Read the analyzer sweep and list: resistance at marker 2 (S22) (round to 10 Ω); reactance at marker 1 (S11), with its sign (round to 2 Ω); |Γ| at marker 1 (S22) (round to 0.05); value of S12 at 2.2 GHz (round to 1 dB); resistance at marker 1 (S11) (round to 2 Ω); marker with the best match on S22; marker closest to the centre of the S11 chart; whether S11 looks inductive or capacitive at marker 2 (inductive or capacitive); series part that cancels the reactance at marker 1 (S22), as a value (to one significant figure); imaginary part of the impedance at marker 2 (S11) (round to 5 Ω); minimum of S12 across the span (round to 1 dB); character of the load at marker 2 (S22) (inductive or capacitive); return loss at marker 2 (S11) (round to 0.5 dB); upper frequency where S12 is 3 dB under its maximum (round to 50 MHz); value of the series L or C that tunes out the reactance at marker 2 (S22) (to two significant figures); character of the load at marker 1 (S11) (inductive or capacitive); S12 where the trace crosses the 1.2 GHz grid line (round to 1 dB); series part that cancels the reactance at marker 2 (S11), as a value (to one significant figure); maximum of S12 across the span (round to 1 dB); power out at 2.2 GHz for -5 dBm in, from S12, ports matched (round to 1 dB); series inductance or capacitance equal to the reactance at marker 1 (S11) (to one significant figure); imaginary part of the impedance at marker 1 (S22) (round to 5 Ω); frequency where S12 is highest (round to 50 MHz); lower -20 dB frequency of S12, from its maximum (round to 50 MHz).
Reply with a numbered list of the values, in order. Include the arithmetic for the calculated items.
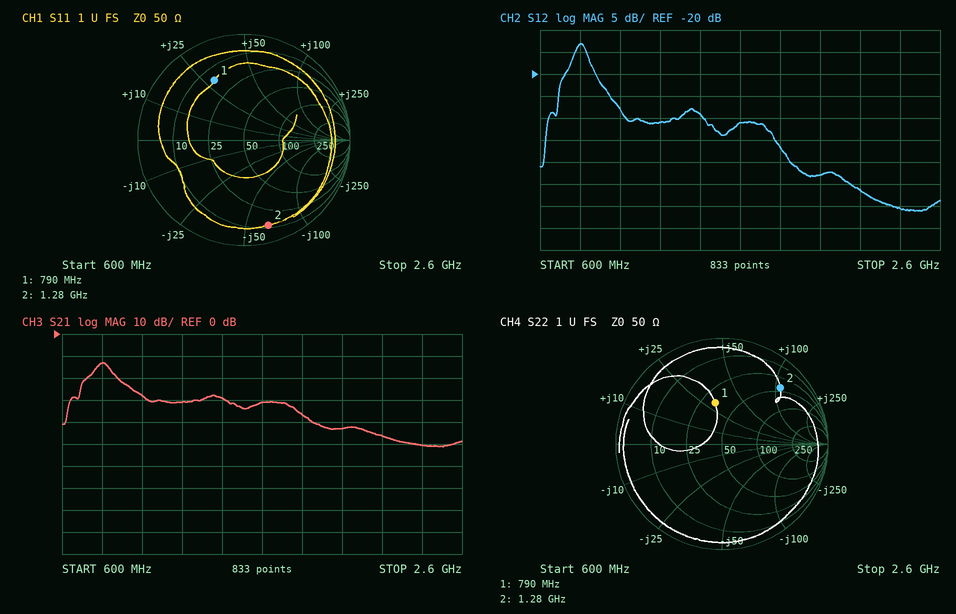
1. 40 Ω
2. +28 Ω
3. 0.40
4. -46 dB
5. 16 Ω
6. marker 1
7. marker 1
8. capacitive
9. C = 1/(2π × 790 MHz × 30 Ω) ≈ 7 pF
10. -65 Ω
11. -51 dB
12. inductive
13. 1.5 dB
14. 850 MHz
15. C = 1/(2π × 1.28 GHz × 110 Ω) ≈ 1.1 pF
16. inductive
17. -31 dB
18. L = 65 Ω/(2π × 1.28 GHz) ≈ 8 nH
19. -13 dB
20. -5 dBm + (-46 dB) = -51 dBm
21. L = 28 Ω/(2π × 790 MHz) ≈ 6 nH
22. +30 Ω
23. 800 MHz
24. 650 MHz
